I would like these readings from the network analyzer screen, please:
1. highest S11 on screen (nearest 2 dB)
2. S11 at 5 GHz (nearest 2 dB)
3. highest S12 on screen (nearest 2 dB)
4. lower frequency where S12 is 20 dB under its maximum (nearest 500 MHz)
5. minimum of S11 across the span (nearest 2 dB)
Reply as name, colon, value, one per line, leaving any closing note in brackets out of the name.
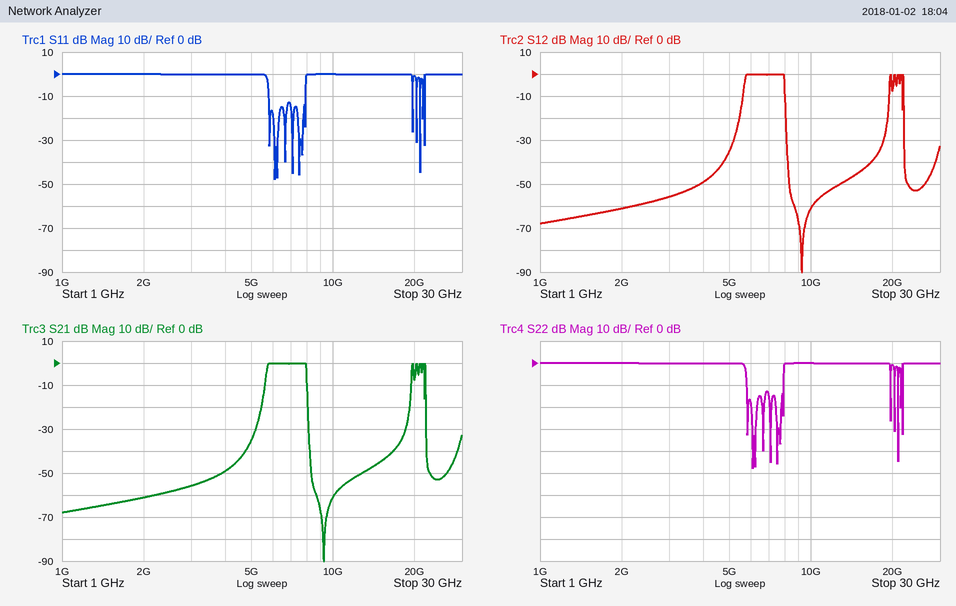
highest S11 on screen: 0 dB
S11 at 5 GHz: 0 dB
highest S12 on screen: 0 dB
lower frequency where S12 is 20 dB under its maximum: 5.5 GHz
minimum of S11 across the span: -48 dB
